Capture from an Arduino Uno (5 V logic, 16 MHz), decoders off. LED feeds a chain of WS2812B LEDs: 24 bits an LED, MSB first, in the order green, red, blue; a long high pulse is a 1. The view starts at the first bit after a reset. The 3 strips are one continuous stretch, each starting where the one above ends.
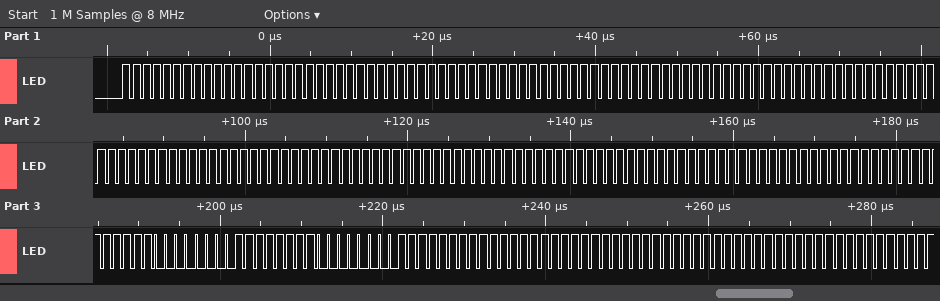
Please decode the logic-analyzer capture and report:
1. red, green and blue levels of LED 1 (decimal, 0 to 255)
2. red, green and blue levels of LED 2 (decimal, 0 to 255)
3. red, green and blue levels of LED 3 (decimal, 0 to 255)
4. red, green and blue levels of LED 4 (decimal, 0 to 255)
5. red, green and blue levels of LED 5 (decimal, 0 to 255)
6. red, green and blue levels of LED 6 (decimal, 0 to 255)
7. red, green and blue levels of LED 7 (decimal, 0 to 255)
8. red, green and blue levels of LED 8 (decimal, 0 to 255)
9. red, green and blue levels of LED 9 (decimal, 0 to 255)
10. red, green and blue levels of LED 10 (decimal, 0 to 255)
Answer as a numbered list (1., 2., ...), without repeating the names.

1. 255, 255, 255
2. 255, 255, 255
3. 255, 255, 255
4. 255, 255, 255
5. 255, 255, 255
6. 255, 255, 255
7. 255, 255, 255
8. 255, 0, 0
9. 255, 255, 255
10. 255, 255, 255
